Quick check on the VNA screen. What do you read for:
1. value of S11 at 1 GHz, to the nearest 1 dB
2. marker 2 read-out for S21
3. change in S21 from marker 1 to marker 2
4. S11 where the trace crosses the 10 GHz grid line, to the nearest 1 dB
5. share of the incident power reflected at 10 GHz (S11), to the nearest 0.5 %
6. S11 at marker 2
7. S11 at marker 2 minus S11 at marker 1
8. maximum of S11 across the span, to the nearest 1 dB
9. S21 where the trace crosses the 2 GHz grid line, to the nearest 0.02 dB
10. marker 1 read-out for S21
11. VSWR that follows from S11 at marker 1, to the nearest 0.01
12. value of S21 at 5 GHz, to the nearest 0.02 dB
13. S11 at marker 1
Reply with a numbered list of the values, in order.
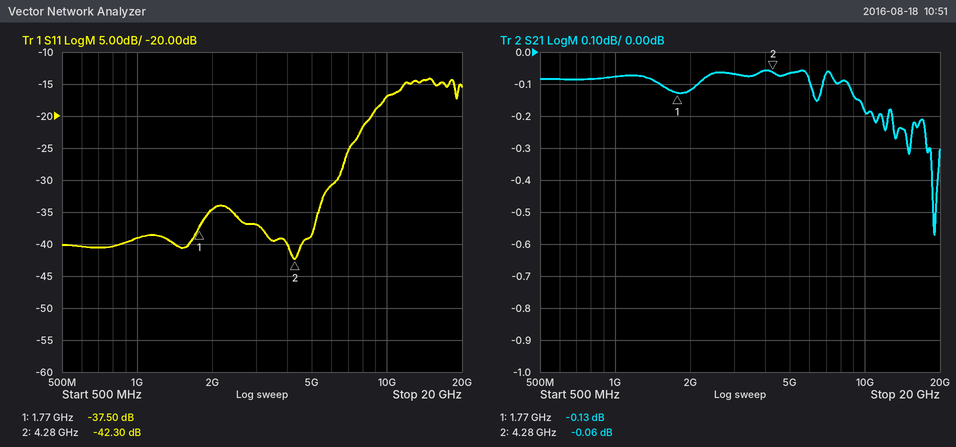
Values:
1. -39 dB
2. -0.06 dB
3. 0.07 dB
4. -17 dB
5. 2.0 %
6. -42.30 dB
7. -4.80 dB
8. -14 dB
9. -0.12 dB
10. -0.13 dB
11. 1.03
12. -0.06 dB
13. -37.50 dB
